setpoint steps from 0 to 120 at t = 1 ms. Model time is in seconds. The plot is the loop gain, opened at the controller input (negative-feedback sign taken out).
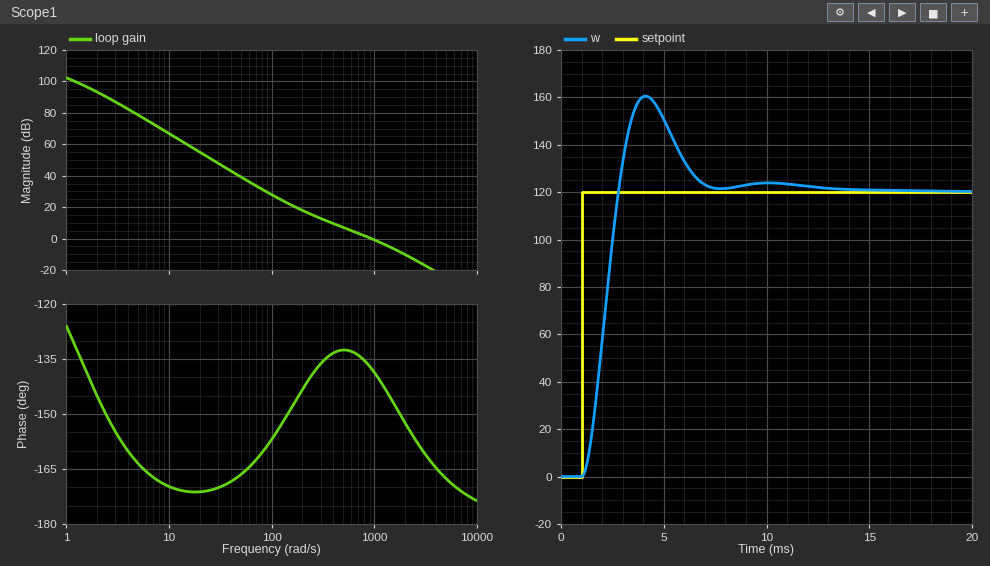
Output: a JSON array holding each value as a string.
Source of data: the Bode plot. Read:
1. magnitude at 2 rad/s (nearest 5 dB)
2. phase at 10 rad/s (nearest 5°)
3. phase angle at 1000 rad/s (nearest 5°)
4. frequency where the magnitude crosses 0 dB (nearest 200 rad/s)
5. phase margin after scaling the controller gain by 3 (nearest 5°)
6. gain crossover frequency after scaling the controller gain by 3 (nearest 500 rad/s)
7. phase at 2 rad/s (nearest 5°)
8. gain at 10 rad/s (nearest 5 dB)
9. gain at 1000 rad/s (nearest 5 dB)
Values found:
["95 dB", "-170°", "-140°", "1000 rad/s", "30°", "2000 rad/s", "-145°", "65 dB", "0 dB"]
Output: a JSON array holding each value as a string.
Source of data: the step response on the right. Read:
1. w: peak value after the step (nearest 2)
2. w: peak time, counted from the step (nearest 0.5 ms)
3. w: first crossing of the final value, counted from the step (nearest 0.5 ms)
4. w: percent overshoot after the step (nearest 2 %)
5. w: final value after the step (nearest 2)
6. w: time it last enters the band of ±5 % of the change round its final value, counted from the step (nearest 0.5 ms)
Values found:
["160", "3.0 ms", "2.0 ms", "34 %", "120", "5.5 ms"]
